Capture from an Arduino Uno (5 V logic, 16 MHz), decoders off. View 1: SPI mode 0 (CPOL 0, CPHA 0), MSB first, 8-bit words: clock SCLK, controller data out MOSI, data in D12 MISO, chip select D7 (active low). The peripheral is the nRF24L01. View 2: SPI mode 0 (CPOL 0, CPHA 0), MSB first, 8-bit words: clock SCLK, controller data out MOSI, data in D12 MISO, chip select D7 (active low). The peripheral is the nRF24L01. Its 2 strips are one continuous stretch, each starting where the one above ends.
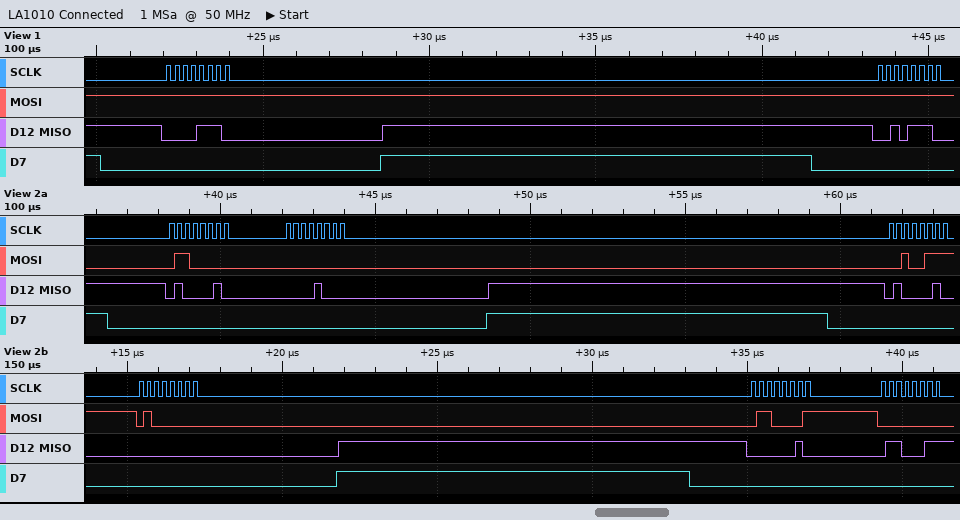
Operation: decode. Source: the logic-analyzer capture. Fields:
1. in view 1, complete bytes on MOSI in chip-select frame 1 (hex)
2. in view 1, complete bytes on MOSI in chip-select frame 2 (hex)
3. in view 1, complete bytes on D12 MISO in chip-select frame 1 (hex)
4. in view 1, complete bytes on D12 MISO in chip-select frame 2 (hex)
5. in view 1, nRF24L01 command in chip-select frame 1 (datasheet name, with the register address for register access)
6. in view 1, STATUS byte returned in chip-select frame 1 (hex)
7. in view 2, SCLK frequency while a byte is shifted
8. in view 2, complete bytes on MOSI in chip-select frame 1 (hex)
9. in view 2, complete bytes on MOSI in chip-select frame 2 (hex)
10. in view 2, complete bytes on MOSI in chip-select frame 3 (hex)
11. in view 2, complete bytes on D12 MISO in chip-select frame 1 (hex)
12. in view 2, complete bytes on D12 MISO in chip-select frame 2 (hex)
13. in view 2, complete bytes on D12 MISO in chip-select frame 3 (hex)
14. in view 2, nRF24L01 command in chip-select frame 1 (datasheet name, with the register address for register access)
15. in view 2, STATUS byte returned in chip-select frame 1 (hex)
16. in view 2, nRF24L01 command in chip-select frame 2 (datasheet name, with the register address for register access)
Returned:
FF
FF
0E
2E
NOP
0x0E
4 MHz
60 00
27 40
61 00
42 08
42 00
02 63
R_RX_PL_WID
0x42
W_REGISTER 0x07
